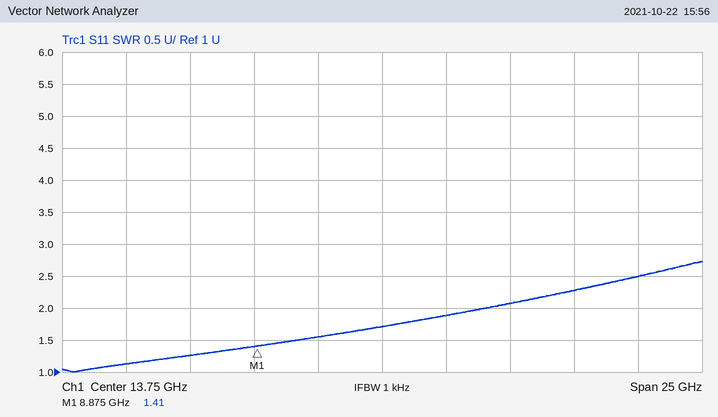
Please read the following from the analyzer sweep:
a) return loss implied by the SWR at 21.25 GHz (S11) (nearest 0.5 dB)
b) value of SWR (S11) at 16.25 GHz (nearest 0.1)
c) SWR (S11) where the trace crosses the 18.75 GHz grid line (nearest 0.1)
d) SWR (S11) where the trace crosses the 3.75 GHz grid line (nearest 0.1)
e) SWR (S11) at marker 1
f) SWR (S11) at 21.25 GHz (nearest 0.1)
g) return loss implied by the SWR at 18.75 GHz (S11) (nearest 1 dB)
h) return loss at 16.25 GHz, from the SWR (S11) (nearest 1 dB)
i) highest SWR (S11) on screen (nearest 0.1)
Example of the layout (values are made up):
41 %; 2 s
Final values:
8.0 dB; 1.9; 2.1; 1.1; 1.41; 2.3; 9 dB; 10 dB; 2.7
